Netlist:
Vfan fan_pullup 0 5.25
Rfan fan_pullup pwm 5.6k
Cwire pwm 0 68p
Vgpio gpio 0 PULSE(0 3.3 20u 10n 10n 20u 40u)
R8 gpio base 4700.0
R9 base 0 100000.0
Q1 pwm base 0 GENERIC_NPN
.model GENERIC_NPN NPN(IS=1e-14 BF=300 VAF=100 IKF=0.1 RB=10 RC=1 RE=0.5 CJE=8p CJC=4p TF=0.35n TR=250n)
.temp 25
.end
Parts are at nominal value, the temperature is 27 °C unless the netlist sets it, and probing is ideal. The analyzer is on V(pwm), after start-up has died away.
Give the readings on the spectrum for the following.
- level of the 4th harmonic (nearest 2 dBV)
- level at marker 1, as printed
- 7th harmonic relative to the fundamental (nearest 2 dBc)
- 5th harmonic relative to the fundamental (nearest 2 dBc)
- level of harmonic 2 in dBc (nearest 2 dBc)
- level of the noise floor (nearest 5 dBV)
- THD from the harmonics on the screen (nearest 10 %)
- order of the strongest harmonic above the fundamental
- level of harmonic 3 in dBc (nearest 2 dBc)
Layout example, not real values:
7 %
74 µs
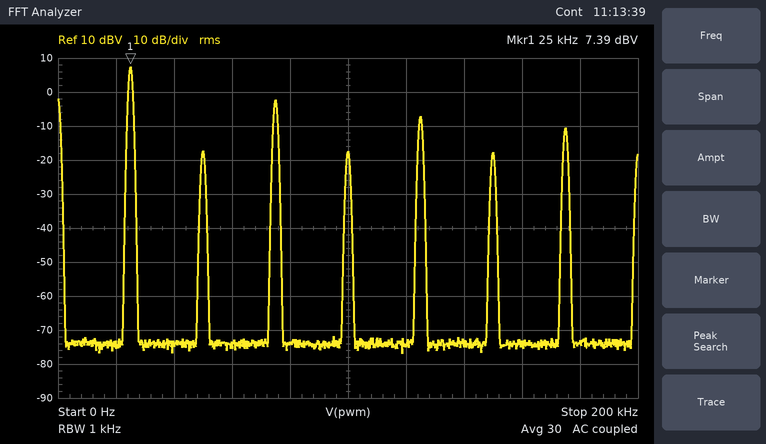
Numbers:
-18 dBV
7.39 dBV
-18 dBc
-14 dBc
-24 dBc
-75 dBV
40 %
3
-10 dBc
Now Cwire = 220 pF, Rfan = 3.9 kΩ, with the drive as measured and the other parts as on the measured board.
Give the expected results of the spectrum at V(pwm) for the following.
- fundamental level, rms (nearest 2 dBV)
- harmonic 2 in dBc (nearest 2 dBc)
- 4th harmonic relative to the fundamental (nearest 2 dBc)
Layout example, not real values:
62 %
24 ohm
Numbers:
8 dBV
-20 dBc
-22 dBc
